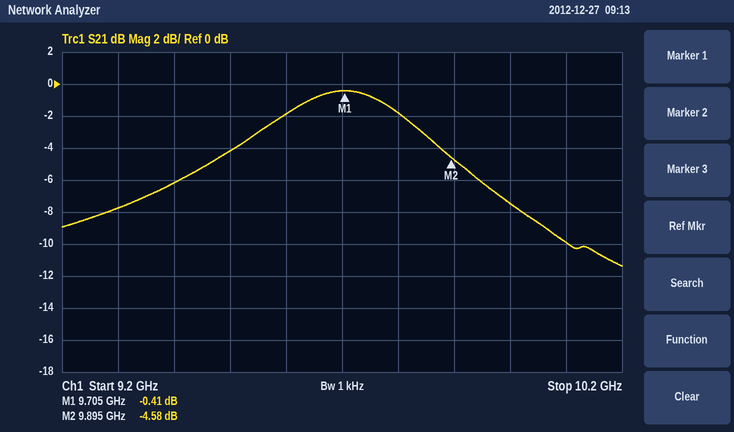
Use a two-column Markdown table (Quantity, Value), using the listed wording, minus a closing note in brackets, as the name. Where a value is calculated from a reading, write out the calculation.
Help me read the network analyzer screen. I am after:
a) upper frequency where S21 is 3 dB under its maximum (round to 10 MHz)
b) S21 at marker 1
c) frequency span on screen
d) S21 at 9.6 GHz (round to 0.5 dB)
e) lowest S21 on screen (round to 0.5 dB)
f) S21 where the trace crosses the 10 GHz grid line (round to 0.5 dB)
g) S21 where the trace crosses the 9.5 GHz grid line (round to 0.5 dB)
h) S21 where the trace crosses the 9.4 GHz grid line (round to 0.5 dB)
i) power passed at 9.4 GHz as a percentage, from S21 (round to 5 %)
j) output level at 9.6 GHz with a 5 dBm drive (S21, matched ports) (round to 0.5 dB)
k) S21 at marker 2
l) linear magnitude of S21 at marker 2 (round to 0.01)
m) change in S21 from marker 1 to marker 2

| Quantity | Value |
|---|---|
| upper frequency where S21 is 3 dB under its maximum | 9.86 GHz |
| S21 at marker 1 | -0.41 dB |
| frequency span on screen | 1 GHz |
| S21 at 9.6 GHz | -2.0 dB |
| lowest S21 on screen | -11.5 dB |
| S21 where the trace crosses the 10 GHz grid line | -7.5 dB |
| S21 where the trace crosses the 9.5 GHz grid line | -4.0 dB |
| S21 where the trace crosses the 9.4 GHz grid line | -6.0 dB |
| power passed at 9.4 GHz as a percentage, from S21 | 10^(-6/10) ≈ 25 % |
| output level at 9.6 GHz with a 5 dBm drive (S21, matched ports) | 5 dBm + (-2.0 dB) = 3.0 dBm |
| S21 at marker 2 | -4.58 dB |
| linear magnitude of S21 at marker 2 | 10^(-4.58/20) ≈ 0.59 |
| change in S21 from marker 1 to marker 2 | -4.58 − (-0.41) = -4.17 dB |
